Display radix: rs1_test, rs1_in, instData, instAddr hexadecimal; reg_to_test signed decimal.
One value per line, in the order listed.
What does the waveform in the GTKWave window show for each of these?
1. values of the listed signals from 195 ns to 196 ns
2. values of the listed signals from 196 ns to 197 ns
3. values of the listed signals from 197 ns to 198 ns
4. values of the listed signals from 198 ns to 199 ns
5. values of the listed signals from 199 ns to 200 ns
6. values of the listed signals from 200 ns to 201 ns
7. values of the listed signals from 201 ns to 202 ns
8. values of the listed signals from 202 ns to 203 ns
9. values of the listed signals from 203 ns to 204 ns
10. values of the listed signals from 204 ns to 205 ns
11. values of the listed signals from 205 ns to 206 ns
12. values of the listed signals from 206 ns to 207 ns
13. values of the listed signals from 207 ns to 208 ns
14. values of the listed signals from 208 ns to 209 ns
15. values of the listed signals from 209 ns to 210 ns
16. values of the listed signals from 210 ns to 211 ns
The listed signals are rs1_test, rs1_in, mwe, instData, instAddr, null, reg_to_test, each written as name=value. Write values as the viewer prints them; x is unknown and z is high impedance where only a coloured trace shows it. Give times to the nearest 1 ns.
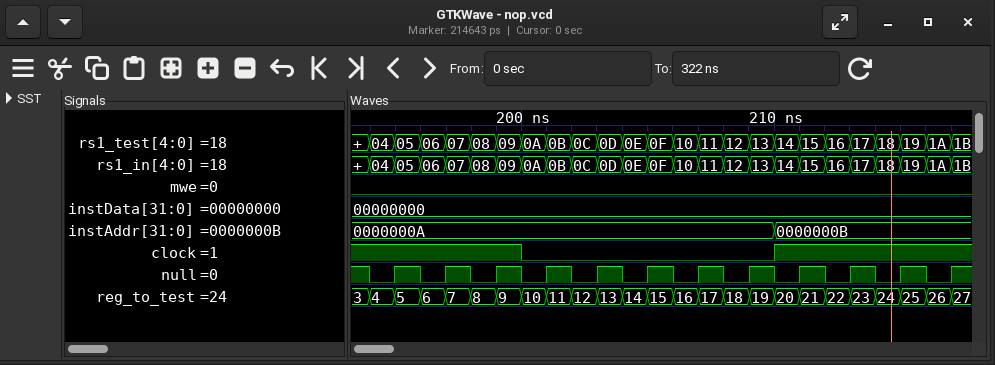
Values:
rs1_test=05, rs1_in=05, mwe=0, instData=00000000, instAddr=0000000A, null=1, reg_to_test=5
rs1_test=06, rs1_in=06, mwe=0, instData=00000000, instAddr=0000000A, null=0, reg_to_test=6
rs1_test=07, rs1_in=07, mwe=0, instData=00000000, instAddr=0000000A, null=1, reg_to_test=7
rs1_test=08, rs1_in=08, mwe=0, instData=00000000, instAddr=0000000A, null=0, reg_to_test=8
rs1_test=09, rs1_in=09, mwe=0, instData=00000000, instAddr=0000000A, null=1, reg_to_test=9
rs1_test=0A, rs1_in=0A, mwe=0, instData=00000000, instAddr=0000000A, null=0, reg_to_test=10
rs1_test=0B, rs1_in=0B, mwe=0, instData=00000000, instAddr=0000000A, null=1, reg_to_test=11
rs1_test=0C, rs1_in=0C, mwe=0, instData=00000000, instAddr=0000000A, null=0, reg_to_test=12
rs1_test=0D, rs1_in=0D, mwe=0, instData=00000000, instAddr=0000000A, null=1, reg_to_test=13
rs1_test=0E, rs1_in=0E, mwe=0, instData=00000000, instAddr=0000000A, null=0, reg_to_test=14
rs1_test=0F, rs1_in=0F, mwe=0, instData=00000000, instAddr=0000000A, null=1, reg_to_test=15
rs1_test=10, rs1_in=10, mwe=0, instData=00000000, instAddr=0000000A, null=0, reg_to_test=16
rs1_test=11, rs1_in=11, mwe=0, instData=00000000, instAddr=0000000A, null=1, reg_to_test=17
rs1_test=12, rs1_in=12, mwe=0, instData=00000000, instAddr=0000000A, null=0, reg_to_test=18
rs1_test=13, rs1_in=13, mwe=0, instData=00000000, instAddr=0000000A, null=1, reg_to_test=19
rs1_test=14, rs1_in=14, mwe=0, instData=00000000, instAddr=0000000B, null=0, reg_to_test=20
